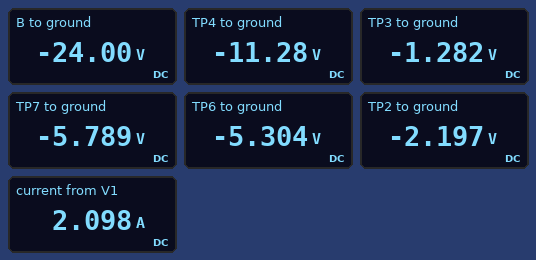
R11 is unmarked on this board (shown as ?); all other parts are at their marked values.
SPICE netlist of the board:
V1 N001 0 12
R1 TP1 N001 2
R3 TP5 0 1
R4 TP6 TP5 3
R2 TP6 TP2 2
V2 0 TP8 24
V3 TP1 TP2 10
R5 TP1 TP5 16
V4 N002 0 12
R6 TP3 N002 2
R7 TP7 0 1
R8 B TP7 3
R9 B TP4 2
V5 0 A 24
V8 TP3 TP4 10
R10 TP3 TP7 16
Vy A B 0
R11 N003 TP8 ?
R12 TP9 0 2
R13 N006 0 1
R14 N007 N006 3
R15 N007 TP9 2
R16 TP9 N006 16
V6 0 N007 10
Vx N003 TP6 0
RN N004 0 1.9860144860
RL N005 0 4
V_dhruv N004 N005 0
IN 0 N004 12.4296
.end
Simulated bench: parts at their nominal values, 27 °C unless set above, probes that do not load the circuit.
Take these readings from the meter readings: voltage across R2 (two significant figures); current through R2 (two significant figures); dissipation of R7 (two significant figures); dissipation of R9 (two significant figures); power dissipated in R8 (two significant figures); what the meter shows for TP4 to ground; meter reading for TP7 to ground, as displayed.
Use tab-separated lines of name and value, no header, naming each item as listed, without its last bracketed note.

voltage across R2	3.1 V
current through R2	1.6 A
dissipation of R7	34 W
dissipation of R9	81 W
power dissipated in R8	110 W
what the meter shows for TP4 to ground	-11.28 V
meter reading for TP7 to ground, as displayed	-5.789 V
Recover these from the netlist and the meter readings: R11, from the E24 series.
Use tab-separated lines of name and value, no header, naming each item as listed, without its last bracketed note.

R11, from the E24 series	6.2 Ω
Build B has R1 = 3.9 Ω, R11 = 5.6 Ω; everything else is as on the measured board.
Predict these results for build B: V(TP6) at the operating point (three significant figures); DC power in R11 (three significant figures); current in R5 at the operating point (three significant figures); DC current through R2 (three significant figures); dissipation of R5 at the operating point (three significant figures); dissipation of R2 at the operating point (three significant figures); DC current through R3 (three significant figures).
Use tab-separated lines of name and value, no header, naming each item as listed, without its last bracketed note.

V(TP6) at the operating point	-6.90 V
DC power in R11	52.2 W
current in R5 at the operating point	434 mA
DC current through R2	1.22 A
dissipation of R5 at the operating point	3.01 W
dissipation of R2 at the operating point	2.98 W
DC current through R3	1.40 A
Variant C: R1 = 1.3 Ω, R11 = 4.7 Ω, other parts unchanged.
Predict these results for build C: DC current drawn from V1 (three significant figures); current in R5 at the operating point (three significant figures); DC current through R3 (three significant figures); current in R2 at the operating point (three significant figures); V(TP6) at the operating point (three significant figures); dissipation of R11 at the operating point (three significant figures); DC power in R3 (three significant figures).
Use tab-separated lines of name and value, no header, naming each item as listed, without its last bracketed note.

DC current drawn from V1	2.78 A
current in R5 at the operating point	590 mA
DC current through R3	1.05 A
current in R2 at the operating point	2.19 A
V(TP6) at the operating point	-5.99 V
dissipation of R11 at the operating point	69.0 W
DC power in R3	1.11 W
